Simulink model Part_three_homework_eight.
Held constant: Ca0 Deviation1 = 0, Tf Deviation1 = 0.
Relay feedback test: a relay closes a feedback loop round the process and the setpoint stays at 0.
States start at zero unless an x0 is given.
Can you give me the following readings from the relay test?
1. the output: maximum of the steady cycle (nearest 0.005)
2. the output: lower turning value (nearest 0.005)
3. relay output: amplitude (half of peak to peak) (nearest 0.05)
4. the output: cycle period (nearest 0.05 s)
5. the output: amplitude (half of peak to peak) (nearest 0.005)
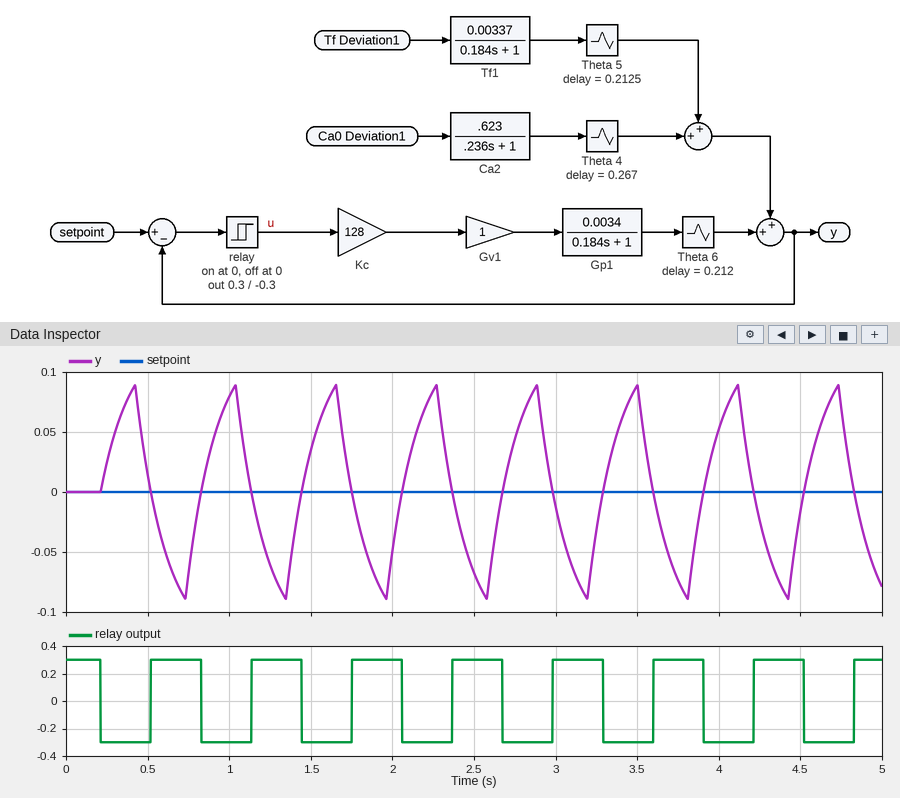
0.090
-0.090
0.30
0.60 s
0.090
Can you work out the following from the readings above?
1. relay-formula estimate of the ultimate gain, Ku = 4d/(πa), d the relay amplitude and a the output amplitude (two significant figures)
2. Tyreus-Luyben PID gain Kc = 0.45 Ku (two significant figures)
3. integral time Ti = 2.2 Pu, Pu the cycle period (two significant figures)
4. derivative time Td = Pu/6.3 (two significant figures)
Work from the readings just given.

4.2
1.9
1.3 s
0.095 s
